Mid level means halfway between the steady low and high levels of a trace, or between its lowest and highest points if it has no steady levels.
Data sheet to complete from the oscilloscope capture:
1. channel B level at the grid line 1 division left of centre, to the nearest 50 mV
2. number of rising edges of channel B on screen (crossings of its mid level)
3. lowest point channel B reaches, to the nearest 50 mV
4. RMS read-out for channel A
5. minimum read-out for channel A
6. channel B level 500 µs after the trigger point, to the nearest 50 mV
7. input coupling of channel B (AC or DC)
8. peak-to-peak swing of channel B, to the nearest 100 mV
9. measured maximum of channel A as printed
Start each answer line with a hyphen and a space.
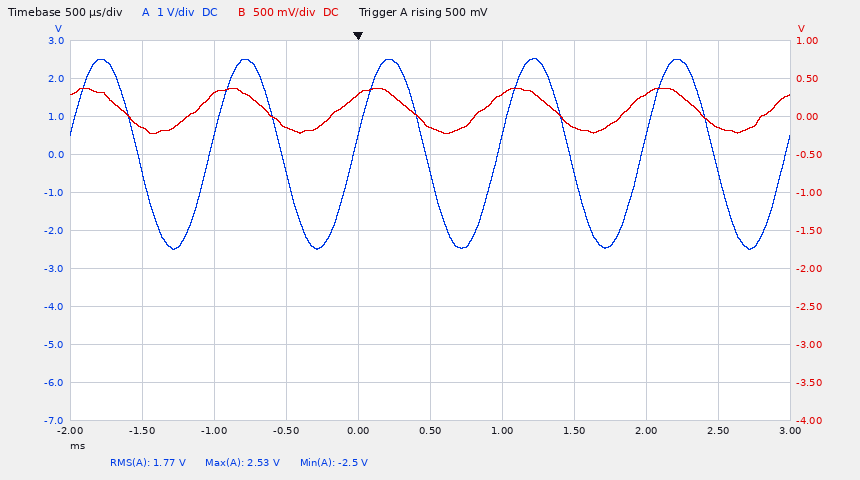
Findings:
- 300 mV
- 5
- -200 mV
- 1.77 V
- -2.5 V
- -150 mV
- DC
- 600 mV
- 2.53 V
